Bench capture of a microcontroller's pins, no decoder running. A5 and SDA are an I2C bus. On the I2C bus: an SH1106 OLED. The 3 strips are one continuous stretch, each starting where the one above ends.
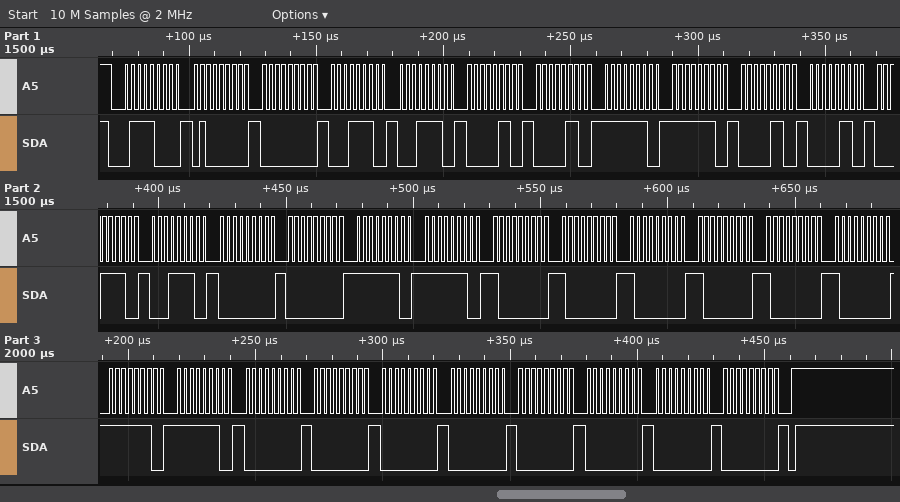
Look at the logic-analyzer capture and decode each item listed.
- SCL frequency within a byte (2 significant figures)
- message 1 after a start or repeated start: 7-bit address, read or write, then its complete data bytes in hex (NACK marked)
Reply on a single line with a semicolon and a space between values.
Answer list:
400 kHz; 0x3C write: 40 00 1E 1E 06 06 FE FE 06 06 1E 1E 00 00 FE FE 80 80 80 80 80 80 FE FE 00 00 00 00 00 00 00 00
